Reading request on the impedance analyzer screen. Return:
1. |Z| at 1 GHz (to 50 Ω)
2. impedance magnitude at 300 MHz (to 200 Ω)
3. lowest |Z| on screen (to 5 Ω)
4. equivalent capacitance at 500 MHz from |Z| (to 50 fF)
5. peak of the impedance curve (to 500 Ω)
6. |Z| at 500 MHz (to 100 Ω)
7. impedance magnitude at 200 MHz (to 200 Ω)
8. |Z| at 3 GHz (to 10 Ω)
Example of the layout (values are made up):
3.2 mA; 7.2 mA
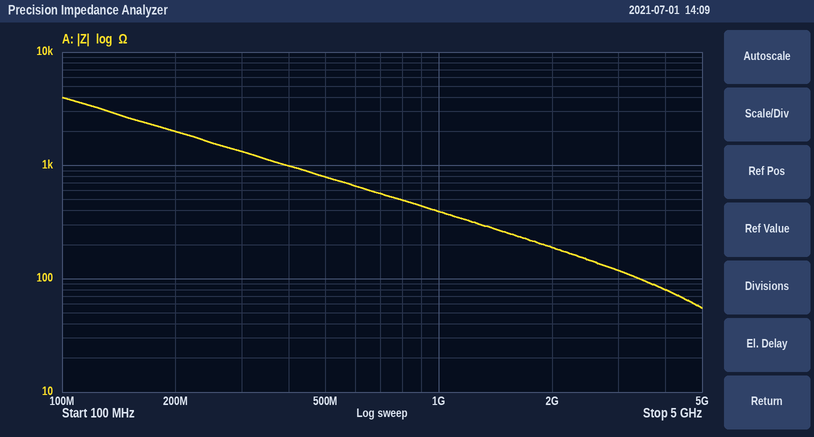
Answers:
400 Ω; 1.4 kΩ; 55 Ω; 400 fF; 4.0 kΩ; 800 Ω; 2.0 kΩ; 120 Ω
